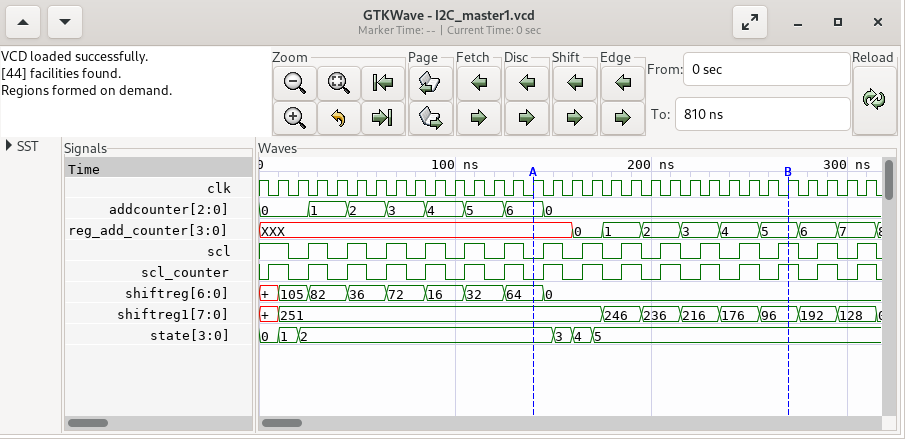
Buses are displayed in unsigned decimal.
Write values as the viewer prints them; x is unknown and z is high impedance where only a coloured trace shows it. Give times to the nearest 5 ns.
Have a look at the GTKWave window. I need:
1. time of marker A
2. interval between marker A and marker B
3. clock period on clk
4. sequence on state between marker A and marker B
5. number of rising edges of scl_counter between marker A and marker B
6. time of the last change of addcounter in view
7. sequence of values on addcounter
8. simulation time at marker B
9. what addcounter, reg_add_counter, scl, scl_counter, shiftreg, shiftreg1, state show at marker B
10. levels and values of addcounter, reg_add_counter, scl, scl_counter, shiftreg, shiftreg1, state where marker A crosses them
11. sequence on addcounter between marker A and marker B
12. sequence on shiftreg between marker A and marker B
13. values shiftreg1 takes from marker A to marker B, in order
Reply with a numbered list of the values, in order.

1. 140 ns
2. 130 ns
3. 10 ns
4. 2, 3, 4, 5
5. 7
6. 145 ns
7. 0, 1, 2, 3, 4, 5, 6, 0
8. 270 ns
9. addcounter=0, reg_add_counter=5, scl=1, scl_counter=1, shiftreg=0, shiftreg1=96, state=5
10. addcounter=6, reg_add_counter=XXX, scl=0, scl_counter=0, shiftreg=64, shiftreg1=251, state=2
11. 6, 0
12. 64, 0
13. 251, 246, 236, 216, 176, 96
